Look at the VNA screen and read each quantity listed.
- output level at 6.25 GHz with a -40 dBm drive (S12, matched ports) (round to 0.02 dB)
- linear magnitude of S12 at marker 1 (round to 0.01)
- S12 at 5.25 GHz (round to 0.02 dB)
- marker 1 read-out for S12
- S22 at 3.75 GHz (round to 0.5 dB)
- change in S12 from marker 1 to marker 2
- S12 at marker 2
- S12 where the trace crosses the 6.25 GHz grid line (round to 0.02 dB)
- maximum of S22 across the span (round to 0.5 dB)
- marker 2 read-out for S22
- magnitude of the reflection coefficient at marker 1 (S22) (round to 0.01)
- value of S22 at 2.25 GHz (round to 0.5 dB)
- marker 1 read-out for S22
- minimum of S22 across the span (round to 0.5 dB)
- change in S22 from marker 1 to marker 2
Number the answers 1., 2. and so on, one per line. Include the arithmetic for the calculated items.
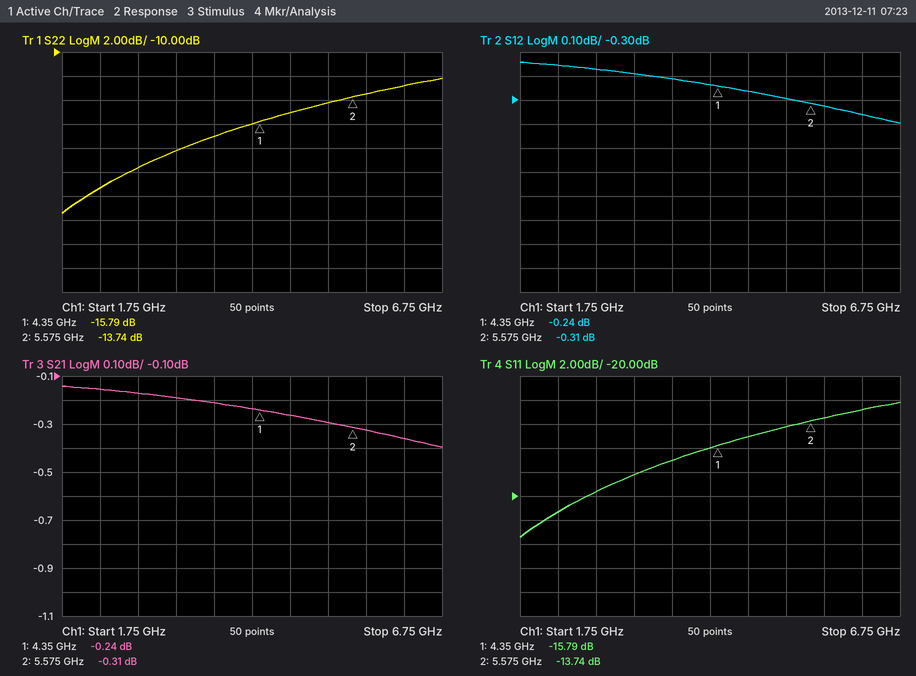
1. -40 dBm + (-0.36 dB) = -40.36 dBm
2. 10^(-0.24/20) ≈ 0.97
3. -0.30 dB
4. -0.24 dB
5. -17.0 dB
6. -0.31 − (-0.24) = -0.07 dB
7. -0.31 dB
8. -0.36 dB
9. -12.0 dB
10. -13.74 dB
11. 10^(-15.79/20) ≈ 0.16
12. -21.5 dB
13. -15.79 dB
14. -23.5 dB
15. -13.74 − (-15.79) = 2.05 dB
